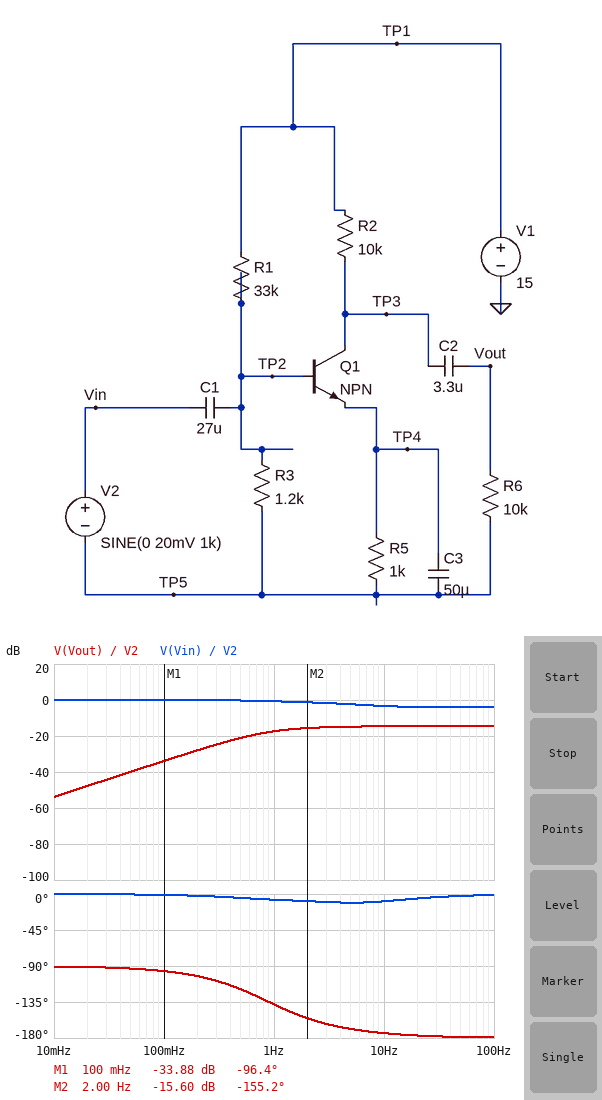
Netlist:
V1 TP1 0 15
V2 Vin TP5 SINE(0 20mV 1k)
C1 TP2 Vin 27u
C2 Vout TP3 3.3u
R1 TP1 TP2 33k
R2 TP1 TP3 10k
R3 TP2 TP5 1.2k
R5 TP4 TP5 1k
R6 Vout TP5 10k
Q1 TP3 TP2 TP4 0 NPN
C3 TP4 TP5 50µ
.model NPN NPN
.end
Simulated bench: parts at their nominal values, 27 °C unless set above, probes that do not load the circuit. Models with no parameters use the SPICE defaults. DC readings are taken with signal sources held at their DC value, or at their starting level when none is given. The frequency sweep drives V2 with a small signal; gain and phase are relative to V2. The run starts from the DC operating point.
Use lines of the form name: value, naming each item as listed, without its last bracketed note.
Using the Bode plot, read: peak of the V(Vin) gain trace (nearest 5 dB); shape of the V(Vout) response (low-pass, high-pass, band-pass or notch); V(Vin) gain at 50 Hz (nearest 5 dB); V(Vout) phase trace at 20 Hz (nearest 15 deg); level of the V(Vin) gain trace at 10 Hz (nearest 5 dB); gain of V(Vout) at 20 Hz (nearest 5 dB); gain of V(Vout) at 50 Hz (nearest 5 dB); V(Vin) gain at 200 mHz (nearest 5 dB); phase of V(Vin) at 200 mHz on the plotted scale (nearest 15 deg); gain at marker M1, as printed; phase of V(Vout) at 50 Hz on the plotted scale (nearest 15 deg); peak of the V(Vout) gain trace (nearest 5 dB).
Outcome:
peak of the V(Vin) gain trace: 0 dB
shape of the V(Vout) response: high-pass
V(Vin) gain at 50 Hz: -5 dB
V(Vout) phase trace at 20 Hz: -180 deg
level of the V(Vin) gain trace at 10 Hz: -5 dB
gain of V(Vout) at 20 Hz: -15 dB
gain of V(Vout) at 50 Hz: -15 dB
V(Vin) gain at 200 mHz: 0 dB
phase of V(Vin) at 200 mHz on the plotted scale: 0 deg
gain at marker M1, as printed: -33.88 dB
phase of V(Vout) at 50 Hz on the plotted scale: -180 deg
peak of the V(Vout) gain trace: -15 dB
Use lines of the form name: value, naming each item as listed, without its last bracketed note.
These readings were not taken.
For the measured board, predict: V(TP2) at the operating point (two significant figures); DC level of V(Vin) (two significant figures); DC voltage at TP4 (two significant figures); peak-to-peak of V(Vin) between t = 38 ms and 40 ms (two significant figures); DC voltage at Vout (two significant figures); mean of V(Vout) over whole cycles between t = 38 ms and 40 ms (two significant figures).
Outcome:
V(TP2) at the operating point: 15 V
DC level of V(Vin): 15 V
DC voltage at TP4: 15 V
peak-to-peak of V(Vin) between t = 38 ms and 40 ms: 25 mV
DC voltage at Vout: 15 V
mean of V(Vout) over whole cycles between t = 38 ms and 40 ms: 15 V
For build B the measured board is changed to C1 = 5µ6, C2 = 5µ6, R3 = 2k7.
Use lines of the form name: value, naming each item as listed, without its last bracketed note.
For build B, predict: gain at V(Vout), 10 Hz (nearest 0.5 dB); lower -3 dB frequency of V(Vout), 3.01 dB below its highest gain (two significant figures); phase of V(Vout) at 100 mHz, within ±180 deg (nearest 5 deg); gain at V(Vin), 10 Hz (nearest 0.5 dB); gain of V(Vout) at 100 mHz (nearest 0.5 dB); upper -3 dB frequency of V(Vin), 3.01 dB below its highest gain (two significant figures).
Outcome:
gain at V(Vout), 10 Hz: -17.5 dB
lower -3 dB frequency of V(Vout), 3.01 dB below its highest gain: 10 Hz
phase of V(Vout) at 100 mHz, within ±180 deg: -100 deg
gain at V(Vin), 10 Hz: -1.5 dB
gain of V(Vout) at 100 mHz: -40.5 dB
upper -3 dB frequency of V(Vin), 3.01 dB below its highest gain: 22 Hz
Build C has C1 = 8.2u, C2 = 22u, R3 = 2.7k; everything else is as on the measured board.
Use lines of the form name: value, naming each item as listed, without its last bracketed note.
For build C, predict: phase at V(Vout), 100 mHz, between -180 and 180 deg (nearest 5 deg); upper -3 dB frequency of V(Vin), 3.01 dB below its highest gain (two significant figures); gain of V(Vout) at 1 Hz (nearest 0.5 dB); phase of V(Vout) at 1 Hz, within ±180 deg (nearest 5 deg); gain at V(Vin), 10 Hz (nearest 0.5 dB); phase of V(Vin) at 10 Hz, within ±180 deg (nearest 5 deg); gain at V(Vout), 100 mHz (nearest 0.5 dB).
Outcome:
phase at V(Vout), 100 mHz, between -180 and 180 deg: -120 deg
upper -3 dB frequency of V(Vin), 3.01 dB below its highest gain: 16 Hz
gain of V(Vout) at 1 Hz: -30.5 dB
phase of V(Vout) at 1 Hz, within ±180 deg: -125 deg
gain at V(Vin), 10 Hz: -2.0 dB
phase of V(Vin) at 10 Hz, within ±180 deg: -15 deg
gain at V(Vout), 100 mHz: -39.0 dB
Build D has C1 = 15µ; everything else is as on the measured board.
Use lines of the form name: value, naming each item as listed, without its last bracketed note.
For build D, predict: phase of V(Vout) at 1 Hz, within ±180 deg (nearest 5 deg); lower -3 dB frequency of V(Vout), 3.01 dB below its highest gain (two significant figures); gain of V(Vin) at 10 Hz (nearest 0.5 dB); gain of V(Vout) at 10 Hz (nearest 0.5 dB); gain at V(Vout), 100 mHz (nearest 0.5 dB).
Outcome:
phase of V(Vout) at 1 Hz, within ±180 deg: -135 deg
lower -3 dB frequency of V(Vout), 3.01 dB below its highest gain: 6.2 Hz
gain of V(Vin) at 10 Hz: -2.0 dB
gain of V(Vout) at 10 Hz: -16.0 dB
gain at V(Vout), 100 mHz: -39.0 dB
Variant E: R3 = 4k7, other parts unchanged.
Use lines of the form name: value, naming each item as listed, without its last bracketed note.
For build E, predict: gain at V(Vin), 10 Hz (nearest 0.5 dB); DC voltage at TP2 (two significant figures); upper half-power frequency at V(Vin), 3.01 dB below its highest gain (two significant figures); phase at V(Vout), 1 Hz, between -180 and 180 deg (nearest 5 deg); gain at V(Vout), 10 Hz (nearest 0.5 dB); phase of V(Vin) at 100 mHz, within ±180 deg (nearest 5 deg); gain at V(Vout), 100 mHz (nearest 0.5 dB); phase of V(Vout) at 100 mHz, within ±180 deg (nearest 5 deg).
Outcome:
gain at V(Vin), 10 Hz: -4.0 dB
DC voltage at TP2: 15 V
upper half-power frequency at V(Vin), 3.01 dB below its highest gain: 780 mHz
phase at V(Vout), 1 Hz, between -180 and 180 deg: -165 deg
gain at V(Vout), 10 Hz: -13.5 dB
phase of V(Vin) at 100 mHz, within ±180 deg: -5 deg
gain at V(Vout), 100 mHz: -22.0 dB
phase of V(Vout) at 100 mHz, within ±180 deg: -100 deg
